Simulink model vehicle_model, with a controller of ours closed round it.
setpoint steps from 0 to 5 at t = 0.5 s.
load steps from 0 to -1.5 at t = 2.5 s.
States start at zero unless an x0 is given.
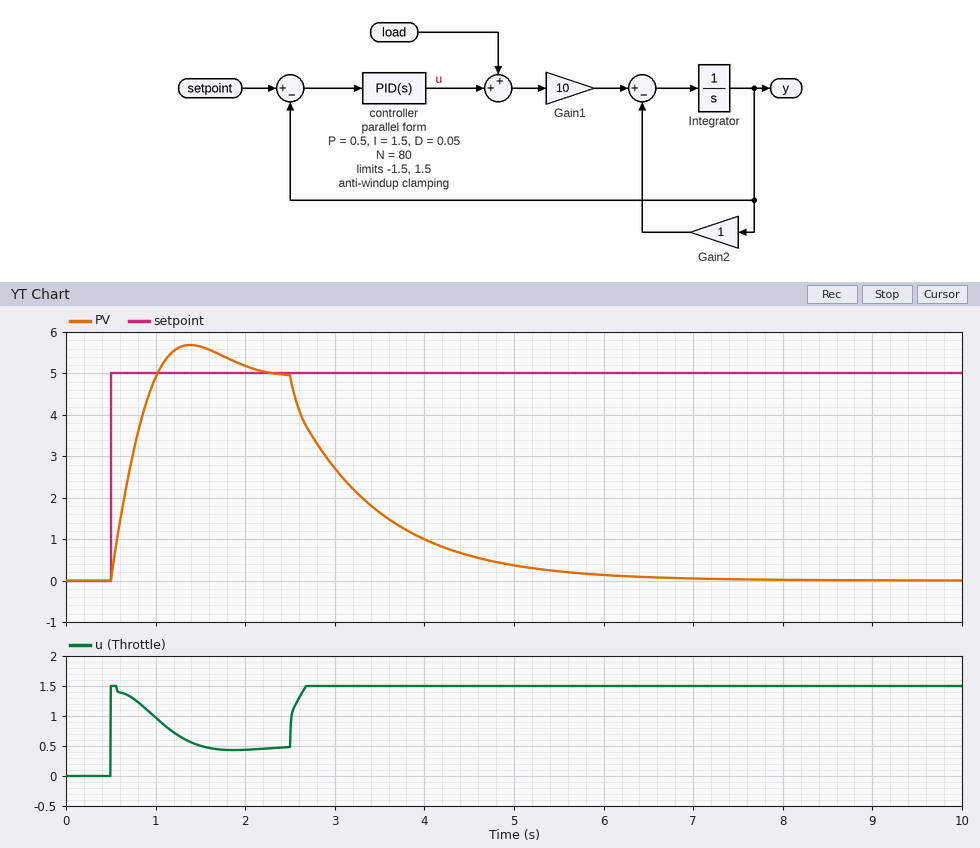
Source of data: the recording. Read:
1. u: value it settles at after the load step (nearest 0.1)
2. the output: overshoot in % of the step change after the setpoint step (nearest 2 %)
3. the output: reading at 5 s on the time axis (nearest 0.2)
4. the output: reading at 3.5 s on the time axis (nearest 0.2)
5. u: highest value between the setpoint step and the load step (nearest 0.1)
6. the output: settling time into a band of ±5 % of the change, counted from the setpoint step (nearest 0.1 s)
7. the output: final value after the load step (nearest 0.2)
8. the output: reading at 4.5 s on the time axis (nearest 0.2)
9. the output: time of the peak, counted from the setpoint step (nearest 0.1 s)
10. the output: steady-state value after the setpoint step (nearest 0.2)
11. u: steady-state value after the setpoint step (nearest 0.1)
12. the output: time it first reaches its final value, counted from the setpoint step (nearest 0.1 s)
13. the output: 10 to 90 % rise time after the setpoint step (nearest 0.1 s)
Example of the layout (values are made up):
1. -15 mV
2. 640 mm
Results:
1. 1.5
2. 14 %
3. 0.4
4. 1.6
5. 1.5
6. 1.4 s
7. 0.0
8. 0.6
9. 0.9 s
10. 5.0
11. 0.5
12. 0.5 s
13. 0.4 s
